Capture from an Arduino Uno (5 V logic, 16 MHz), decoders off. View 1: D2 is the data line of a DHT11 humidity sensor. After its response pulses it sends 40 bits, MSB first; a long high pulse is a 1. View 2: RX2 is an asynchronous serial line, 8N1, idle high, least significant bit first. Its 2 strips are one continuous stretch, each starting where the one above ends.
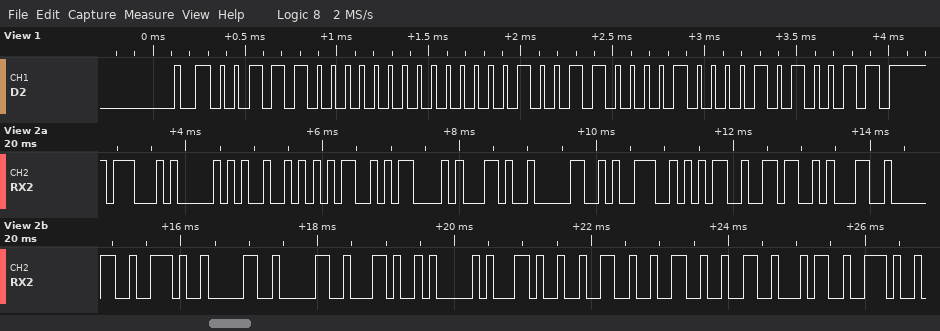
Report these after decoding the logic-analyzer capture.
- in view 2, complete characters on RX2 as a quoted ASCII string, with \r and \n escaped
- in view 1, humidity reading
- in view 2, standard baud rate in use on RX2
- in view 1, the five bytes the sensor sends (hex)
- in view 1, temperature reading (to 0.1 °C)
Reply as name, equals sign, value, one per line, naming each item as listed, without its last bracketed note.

in view 2, complete characters on RX2 as a quoted ASCII string, with \r and \n escaped = "GPRMC,095610.00,A,2224."
in view 1, humidity reading = 56 %
in view 2, standard baud rate in use on RX2 = 9600 baud
in view 1, the five bytes the sensor sends = 38 00 13 08 53
in view 1, temperature reading = 19.8 °C
